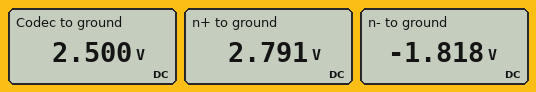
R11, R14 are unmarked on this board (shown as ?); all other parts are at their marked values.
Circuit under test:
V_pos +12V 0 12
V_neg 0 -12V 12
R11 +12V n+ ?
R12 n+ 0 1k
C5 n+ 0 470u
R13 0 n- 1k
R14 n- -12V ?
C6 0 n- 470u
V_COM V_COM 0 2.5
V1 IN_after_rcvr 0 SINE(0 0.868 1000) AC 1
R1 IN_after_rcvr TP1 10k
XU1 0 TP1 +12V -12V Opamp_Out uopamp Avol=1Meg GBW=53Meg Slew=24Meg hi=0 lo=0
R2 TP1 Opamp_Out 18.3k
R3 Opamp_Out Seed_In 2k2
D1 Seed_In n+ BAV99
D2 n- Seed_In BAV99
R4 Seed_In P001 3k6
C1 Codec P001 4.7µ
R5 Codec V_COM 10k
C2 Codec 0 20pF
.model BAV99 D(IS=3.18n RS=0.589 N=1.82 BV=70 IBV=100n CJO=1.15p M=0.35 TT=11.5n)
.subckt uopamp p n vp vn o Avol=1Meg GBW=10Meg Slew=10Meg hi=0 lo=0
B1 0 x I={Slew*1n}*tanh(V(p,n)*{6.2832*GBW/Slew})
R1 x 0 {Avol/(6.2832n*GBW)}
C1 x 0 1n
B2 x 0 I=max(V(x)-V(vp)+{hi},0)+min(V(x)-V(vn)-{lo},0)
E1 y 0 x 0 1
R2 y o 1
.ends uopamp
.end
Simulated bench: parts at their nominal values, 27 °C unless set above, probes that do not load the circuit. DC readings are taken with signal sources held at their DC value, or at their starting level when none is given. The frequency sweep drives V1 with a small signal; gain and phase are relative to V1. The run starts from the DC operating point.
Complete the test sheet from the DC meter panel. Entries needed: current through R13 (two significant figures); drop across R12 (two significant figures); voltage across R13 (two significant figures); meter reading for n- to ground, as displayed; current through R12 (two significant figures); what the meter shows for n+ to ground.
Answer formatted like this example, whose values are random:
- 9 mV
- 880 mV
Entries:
- 1.8 mA
- 2.8 V
- 1.8 V
- -1.818 V
- 2.8 mA
- 2.791 V
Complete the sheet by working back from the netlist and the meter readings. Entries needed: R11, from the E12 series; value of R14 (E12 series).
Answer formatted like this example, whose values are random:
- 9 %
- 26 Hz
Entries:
- 3.3 kΩ
- 5.6 kΩ
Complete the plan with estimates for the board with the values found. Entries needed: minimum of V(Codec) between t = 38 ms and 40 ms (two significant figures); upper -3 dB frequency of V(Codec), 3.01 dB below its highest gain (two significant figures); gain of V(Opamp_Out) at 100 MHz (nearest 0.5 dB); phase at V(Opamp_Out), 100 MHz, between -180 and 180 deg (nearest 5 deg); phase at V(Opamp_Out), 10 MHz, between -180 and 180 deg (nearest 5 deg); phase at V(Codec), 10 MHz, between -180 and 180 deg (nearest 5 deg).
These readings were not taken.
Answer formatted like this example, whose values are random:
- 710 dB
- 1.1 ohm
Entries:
- 1.5 V
- 2.1 MHz
- -9.5 dB
- 100 deg
- 150 deg
- 65 deg
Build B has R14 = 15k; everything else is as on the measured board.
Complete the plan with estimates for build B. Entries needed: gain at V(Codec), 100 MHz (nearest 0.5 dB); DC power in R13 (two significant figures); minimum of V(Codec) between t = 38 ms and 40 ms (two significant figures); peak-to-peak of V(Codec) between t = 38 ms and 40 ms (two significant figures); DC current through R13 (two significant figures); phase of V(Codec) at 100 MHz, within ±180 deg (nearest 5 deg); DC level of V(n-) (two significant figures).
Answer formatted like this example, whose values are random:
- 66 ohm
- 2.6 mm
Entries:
- -51.5 dB
- 560 µW
- 1.6 V
- 1.9 V
- 750 µA
- -45 deg
- -750 mV
